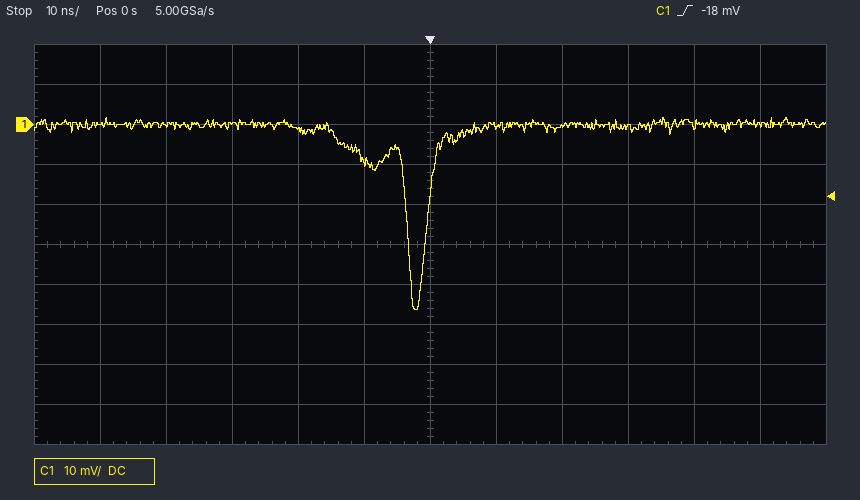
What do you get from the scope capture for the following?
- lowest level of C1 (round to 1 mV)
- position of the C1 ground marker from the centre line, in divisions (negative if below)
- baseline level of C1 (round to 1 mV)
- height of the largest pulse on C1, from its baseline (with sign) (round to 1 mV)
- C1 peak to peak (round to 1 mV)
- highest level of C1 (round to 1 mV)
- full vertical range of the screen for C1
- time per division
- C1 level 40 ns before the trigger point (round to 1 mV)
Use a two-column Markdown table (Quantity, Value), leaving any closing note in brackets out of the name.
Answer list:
| Quantity | Value |
|---|---|
| lowest level of C1 | -46 mV |
| position of the C1 ground marker from the centre line, in divisions | +3.0 div |
| baseline level of C1 | 0 mV |
| height of the largest pulse on C1, from its baseline (with sign) | -46 mV |
| C1 peak to peak | 48 mV |
| highest level of C1 | 2 mV |
| full vertical range of the screen for C1 | 100 mV |
| time per division | 10 ns |
| C1 level 40 ns before the trigger point | 0 mV |
